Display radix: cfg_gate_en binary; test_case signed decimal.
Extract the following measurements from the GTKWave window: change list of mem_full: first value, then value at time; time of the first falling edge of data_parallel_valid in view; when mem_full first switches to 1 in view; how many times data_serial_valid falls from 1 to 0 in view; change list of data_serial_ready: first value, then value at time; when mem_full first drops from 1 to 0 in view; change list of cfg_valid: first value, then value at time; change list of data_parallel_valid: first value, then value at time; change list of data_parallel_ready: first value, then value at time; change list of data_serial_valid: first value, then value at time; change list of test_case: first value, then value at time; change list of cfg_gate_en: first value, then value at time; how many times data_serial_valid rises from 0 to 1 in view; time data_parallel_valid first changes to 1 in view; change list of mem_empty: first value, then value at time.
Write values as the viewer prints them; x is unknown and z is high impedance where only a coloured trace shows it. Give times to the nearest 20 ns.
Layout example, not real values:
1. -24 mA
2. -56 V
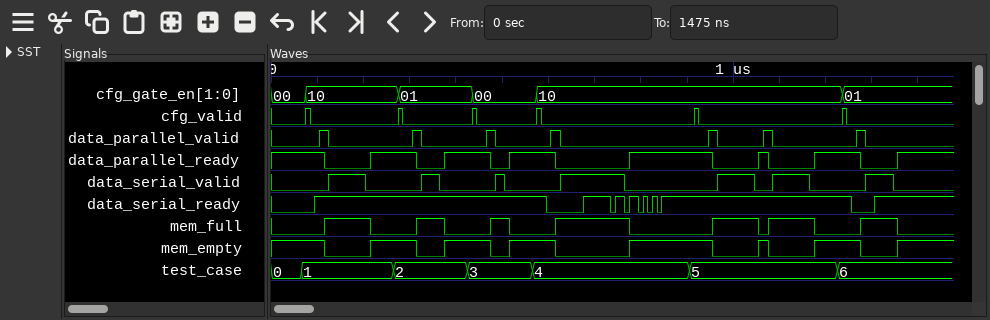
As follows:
1. 0, 1 at 120 ns, 0 at 220 ns, 1 at 320 ns, 0 at 380 ns, 1 at 480 ns, 0 at 520 ns, 1 at 620 ns, 0 at 780 ns, 1 at 960 ns, 0 at 1060 ns, 1 at 1080 ns, 0 at 1180 ns, 1 at 1280 ns, 0 at 1360 ns
2. 120 ns
3. 120 ns
4. 7
5. 0, 1 at 100 ns, 0 at 600 ns, 1 at 680 ns, 0 at 740 ns, 1 at 740 ns, 0 at 760 ns, 1 at 780 ns, 0 at 800 ns, 1 at 800 ns, 0 at 820 ns, 1 at 820 ns, 0 at 840 ns, 1 at 840 ns, 0 at 1260 ns, 1 at 1300 ns
6. 220 ns
7. 0, 1 at 80 ns, 0 at 80 ns, 1 at 280 ns, 0 at 280 ns, 1 at 440 ns, 0 at 440 ns, 1 at 580 ns, 0 at 580 ns, 1 at 920 ns, 0 at 920 ns, 1 at 1240 ns, 0 at 1240 ns
8. 0, 1 at 100 ns, 0 at 120 ns, 1 at 300 ns, 0 at 320 ns, 1 at 460 ns, 0 at 480 ns, 1 at 600 ns, 0 at 620 ns, 1 at 940 ns, 0 at 960 ns, 1 at 1060 ns, 0 at 1080 ns, 1 at 1260 ns, 0 at 1280 ns
9. 1, 0 at 120 ns, 1 at 220 ns, 0 at 320 ns, 1 at 380 ns, 0 at 480 ns, 1 at 520 ns, 0 at 620 ns, 1 at 780 ns, 0 at 960 ns, 1 at 1060 ns, 0 at 1080 ns, 1 at 1180 ns, 0 at 1280 ns, 1 at 1360 ns
10. 0, 1 at 120 ns, 0 at 200 ns, 1 at 320 ns, 0 at 360 ns, 1 at 480 ns, 0 at 500 ns, 1 at 620 ns, 0 at 760 ns, 1 at 960 ns, 0 at 1040 ns, 1 at 1080 ns, 0 at 1160 ns, 1 at 1280 ns, 0 at 1340 ns
11. 0, 1 at 60 ns, 2 at 260 ns, 3 at 420 ns, 4 at 560 ns, 5 at 900 ns, 6 at 1220 ns
12. 00, 10 at 80 ns, 01 at 280 ns, 00 at 440 ns, 10 at 580 ns, 01 at 1240 ns
13. 7
14. 100 ns
15. 1, 0 at 120 ns, 1 at 220 ns, 0 at 320 ns, 1 at 380 ns, 0 at 480 ns, 1 at 520 ns, 0 at 620 ns, 1 at 780 ns, 0 at 960 ns, 1 at 1060 ns, 0 at 1080 ns, 1 at 1180 ns, 0 at 1280 ns, 1 at 1360 ns
